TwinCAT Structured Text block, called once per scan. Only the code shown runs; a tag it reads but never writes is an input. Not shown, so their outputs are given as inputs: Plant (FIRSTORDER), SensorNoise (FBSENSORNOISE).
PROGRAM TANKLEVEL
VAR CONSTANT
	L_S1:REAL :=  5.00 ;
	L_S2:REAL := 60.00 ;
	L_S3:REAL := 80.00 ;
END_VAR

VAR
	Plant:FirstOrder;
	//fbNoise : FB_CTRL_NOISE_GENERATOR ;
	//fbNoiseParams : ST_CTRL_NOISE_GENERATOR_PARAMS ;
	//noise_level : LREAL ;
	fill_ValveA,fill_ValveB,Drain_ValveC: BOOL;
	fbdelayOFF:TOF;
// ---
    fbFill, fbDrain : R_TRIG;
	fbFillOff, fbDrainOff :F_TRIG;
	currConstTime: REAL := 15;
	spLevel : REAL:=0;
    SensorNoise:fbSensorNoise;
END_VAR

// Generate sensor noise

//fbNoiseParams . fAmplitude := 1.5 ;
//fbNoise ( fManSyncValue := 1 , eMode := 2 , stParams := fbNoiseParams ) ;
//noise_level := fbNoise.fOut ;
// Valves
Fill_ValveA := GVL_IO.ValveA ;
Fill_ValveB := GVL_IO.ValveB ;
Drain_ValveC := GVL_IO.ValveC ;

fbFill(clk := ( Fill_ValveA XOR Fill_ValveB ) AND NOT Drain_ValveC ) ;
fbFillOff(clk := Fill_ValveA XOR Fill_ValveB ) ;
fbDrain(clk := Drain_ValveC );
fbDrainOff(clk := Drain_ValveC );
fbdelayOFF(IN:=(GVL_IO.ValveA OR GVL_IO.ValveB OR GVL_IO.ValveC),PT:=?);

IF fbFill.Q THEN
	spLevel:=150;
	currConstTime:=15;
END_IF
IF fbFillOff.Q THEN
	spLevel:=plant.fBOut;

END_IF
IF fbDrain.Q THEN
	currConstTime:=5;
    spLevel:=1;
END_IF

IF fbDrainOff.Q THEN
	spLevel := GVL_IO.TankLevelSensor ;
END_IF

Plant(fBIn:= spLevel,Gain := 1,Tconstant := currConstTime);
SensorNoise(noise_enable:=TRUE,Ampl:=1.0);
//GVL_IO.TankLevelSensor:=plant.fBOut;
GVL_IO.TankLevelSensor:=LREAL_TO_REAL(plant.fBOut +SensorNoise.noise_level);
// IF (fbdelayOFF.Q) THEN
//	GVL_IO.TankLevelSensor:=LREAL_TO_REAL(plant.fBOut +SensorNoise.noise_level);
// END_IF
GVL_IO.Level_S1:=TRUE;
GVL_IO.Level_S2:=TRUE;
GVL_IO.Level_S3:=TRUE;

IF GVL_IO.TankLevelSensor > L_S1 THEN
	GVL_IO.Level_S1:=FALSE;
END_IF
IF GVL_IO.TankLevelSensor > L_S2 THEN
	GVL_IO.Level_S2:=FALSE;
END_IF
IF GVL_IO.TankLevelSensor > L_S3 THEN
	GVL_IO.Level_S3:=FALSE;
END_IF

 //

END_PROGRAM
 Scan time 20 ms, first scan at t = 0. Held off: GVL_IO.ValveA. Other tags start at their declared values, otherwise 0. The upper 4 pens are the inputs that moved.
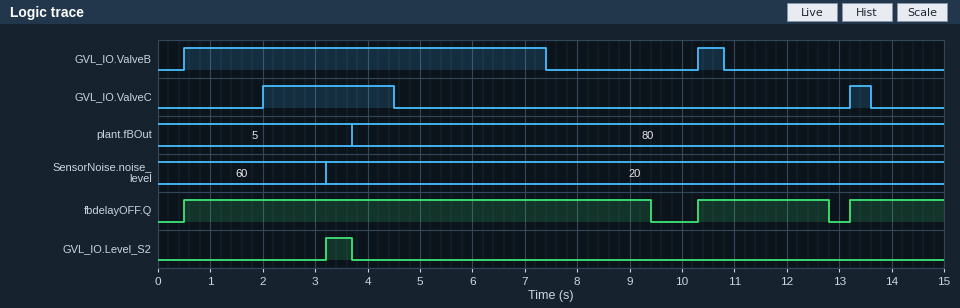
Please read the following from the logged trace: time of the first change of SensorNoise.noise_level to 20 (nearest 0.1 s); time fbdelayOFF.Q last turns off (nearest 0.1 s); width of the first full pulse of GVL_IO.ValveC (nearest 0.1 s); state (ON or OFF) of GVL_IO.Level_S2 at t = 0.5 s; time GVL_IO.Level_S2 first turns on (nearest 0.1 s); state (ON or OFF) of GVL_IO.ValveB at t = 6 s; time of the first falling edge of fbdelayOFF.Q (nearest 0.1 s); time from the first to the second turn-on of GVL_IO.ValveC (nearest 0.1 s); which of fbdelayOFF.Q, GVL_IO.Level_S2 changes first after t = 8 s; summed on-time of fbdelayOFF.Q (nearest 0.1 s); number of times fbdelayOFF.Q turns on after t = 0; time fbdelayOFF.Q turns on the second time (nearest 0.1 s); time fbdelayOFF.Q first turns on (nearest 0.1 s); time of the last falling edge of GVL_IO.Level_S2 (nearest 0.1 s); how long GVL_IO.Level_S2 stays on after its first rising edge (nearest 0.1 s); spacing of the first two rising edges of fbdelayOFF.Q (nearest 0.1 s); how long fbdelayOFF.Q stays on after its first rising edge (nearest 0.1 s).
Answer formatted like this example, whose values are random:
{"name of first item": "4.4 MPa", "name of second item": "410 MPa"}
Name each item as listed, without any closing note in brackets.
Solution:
{"time of the first change of SensorNoise.noise_level to 20": "3.2 s", "time fbdelayOFF.Q last turns off": "12.8 s", "width of the first full pulse of GVL_IO.ValveC": "2.5 s", "state (ON or OFF) of GVL_IO.Level_S2 at t = 0.5 s": "OFF", "time GVL_IO.Level_S2 first turns on": "3.2 s", "state (ON or OFF) of GVL_IO.ValveB at t = 6 s": "ON", "time of the first falling edge of fbdelayOFF.Q": "9.4 s", "time from the first to the second turn-on of GVL_IO.ValveC": "11.2 s", "which of fbdelayOFF.Q, GVL_IO.Level_S2 changes first after t = 8 s": "fbdelayOFF.Q", "summed on-time of fbdelayOFF.Q": "13.2 s", "number of times fbdelayOFF.Q turns on after t = 0": "3", "time fbdelayOFF.Q turns on the second time": "10.3 s", "time fbdelayOFF.Q first turns on": "0.5 s", "time of the last falling edge of GVL_IO.Level_S2": "3.7 s", "how long GVL_IO.Level_S2 stays on after its first rising edge": "0.5 s", "spacing of the first two rising edges of fbdelayOFF.Q": "9.8 s", "how long fbdelayOFF.Q stays on after its first rising edge": "8.9 s"}
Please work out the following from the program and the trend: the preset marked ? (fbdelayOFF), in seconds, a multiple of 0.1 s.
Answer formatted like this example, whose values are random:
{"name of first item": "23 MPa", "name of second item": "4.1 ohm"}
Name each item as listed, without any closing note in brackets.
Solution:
{"the preset marked ? (fbdelayOFF), in seconds, a multiple of 0.1 s": "2.0 s"}
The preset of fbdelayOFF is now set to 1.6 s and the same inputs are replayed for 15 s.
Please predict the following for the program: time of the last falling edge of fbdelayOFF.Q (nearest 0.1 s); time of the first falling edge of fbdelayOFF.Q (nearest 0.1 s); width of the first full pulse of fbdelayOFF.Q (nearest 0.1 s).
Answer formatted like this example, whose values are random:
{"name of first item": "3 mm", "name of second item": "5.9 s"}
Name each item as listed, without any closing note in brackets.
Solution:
{"time of the last falling edge of fbdelayOFF.Q": "12.4 s", "time of the first falling edge of fbdelayOFF.Q": "9.0 s", "width of the first full pulse of fbdelayOFF.Q": "8.5 s"}
